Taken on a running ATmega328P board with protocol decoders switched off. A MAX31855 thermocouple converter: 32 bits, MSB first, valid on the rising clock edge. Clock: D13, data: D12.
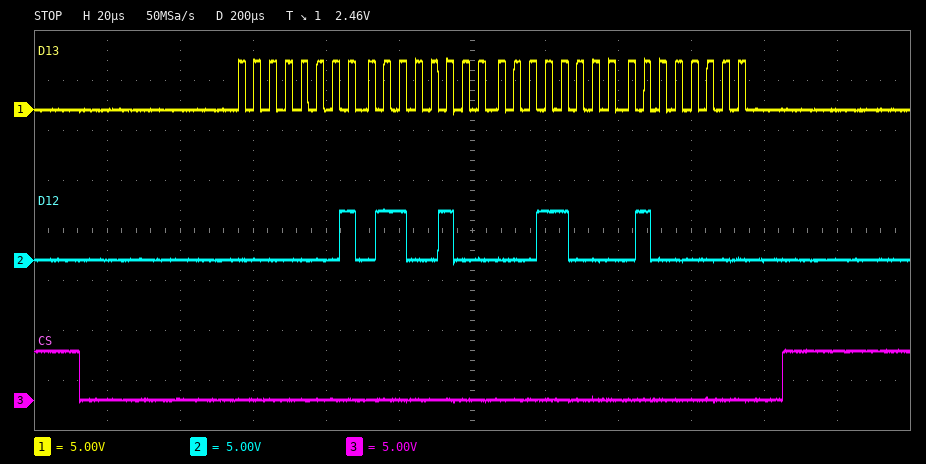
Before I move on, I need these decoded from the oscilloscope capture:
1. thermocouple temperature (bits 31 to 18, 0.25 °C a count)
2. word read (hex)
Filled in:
22.25 °C
0x01641840
